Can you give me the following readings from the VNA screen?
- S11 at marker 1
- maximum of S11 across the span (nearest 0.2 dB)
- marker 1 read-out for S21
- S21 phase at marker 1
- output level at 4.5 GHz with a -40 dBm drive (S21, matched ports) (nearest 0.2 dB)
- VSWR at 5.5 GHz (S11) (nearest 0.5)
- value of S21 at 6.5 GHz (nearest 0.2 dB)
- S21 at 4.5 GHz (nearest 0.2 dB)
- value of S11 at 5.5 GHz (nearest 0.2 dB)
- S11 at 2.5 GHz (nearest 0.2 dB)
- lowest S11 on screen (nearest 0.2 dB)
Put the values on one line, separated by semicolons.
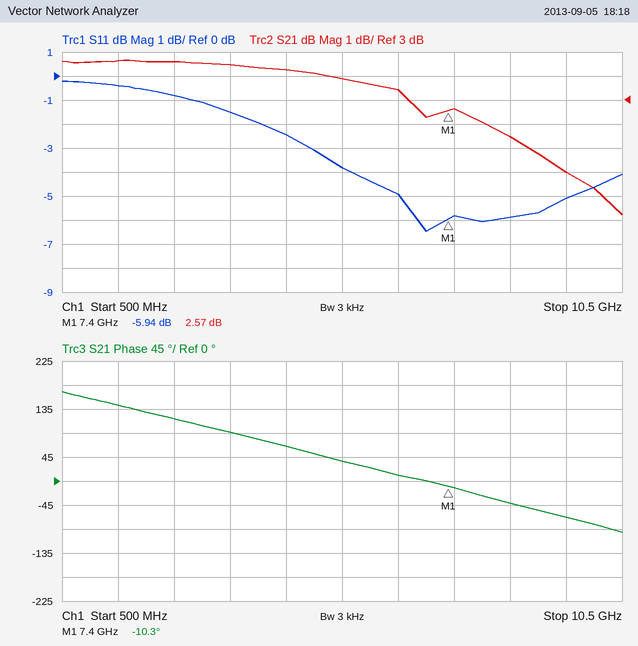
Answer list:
-5.94 dB; -0.2 dB; 2.57 dB; -10.3°; -35.8 dBm; 4.5; 3.4 dB; 4.2 dB; -3.8 dB; -0.8 dB; -6.4 dB
